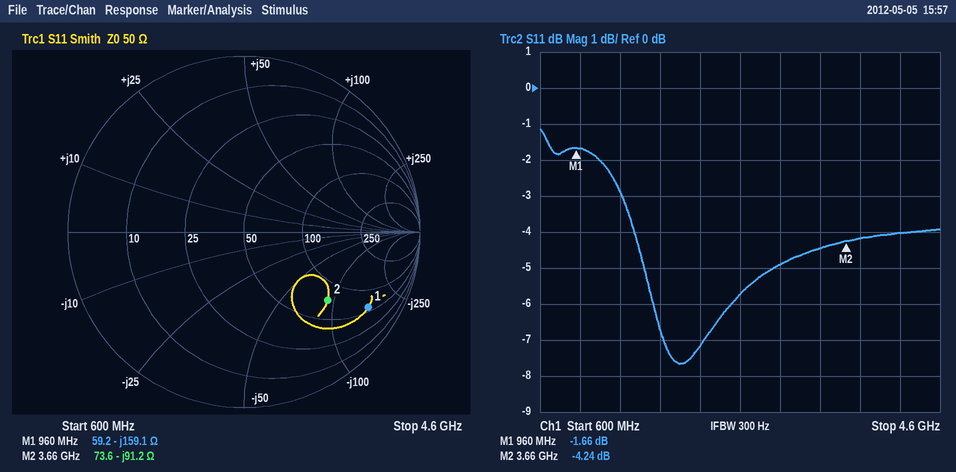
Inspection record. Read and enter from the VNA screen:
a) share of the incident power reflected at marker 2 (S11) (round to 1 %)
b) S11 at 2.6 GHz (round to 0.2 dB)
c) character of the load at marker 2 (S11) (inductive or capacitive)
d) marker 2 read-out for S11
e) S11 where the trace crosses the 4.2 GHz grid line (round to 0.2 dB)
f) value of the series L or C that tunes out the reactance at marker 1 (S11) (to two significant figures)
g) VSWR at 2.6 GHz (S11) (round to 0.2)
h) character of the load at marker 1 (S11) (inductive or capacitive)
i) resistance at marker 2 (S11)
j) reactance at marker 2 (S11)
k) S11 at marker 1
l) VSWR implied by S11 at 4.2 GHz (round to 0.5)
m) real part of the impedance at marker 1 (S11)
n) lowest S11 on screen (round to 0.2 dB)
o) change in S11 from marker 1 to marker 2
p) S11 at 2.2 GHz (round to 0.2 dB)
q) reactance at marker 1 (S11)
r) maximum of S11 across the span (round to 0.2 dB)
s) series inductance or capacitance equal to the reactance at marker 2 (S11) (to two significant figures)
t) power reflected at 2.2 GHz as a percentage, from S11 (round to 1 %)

38 %
-5.8 dB
capacitive
-4.24 dB
-4.0 dB
26 nH
3.2
capacitive
73.6 Ω
-91.2 Ω
-1.66 dB
4.5
59.2 Ω
-7.6 dB
-2.58 dB
-7.2 dB
-159.1 Ω
-1.2 dB
480 fF
19 %
